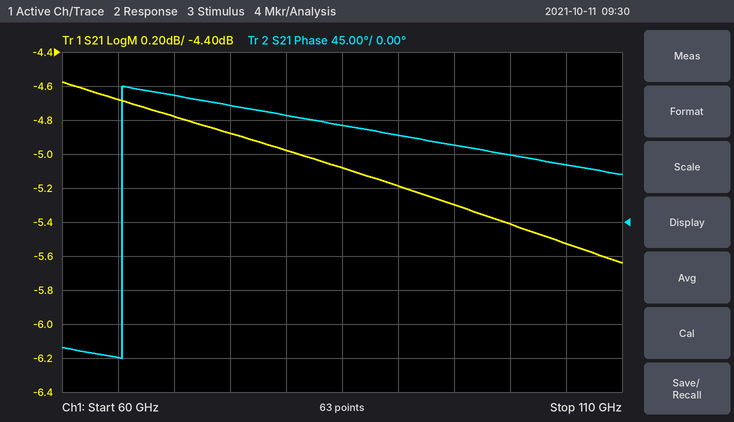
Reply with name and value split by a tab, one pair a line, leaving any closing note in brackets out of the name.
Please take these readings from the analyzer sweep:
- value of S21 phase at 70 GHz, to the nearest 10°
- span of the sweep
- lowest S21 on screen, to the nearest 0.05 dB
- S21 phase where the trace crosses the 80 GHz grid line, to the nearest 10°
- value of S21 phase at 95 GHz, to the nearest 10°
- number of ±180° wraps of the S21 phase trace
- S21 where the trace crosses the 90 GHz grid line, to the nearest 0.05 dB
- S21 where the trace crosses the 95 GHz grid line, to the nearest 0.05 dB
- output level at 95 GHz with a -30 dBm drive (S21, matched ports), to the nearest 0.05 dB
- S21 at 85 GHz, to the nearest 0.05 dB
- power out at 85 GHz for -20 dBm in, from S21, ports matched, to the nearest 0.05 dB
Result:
value of S21 phase at 70 GHz, to the nearest 10°	170°
span of the sweep	50 GHz
lowest S21 on screen, to the nearest 0.05 dB	-5.65 dB
S21 phase where the trace crosses the 80 GHz grid line, to the nearest 10°	140°
value of S21 phase at 95 GHz, to the nearest 10°	100°
number of ±180° wraps of the S21 phase trace	1
S21 where the trace crosses the 90 GHz grid line, to the nearest 0.05 dB	-5.20 dB
S21 where the trace crosses the 95 GHz grid line, to the nearest 0.05 dB	-5.30 dB
output level at 95 GHz with a -30 dBm drive (S21, matched ports), to the nearest 0.05 dB	-35.30 dBm
S21 at 85 GHz, to the nearest 0.05 dB	-5.10 dB
power out at 85 GHz for -20 dBm in, from S21, ports matched, to the nearest 0.05 dB	-25.10 dBm
